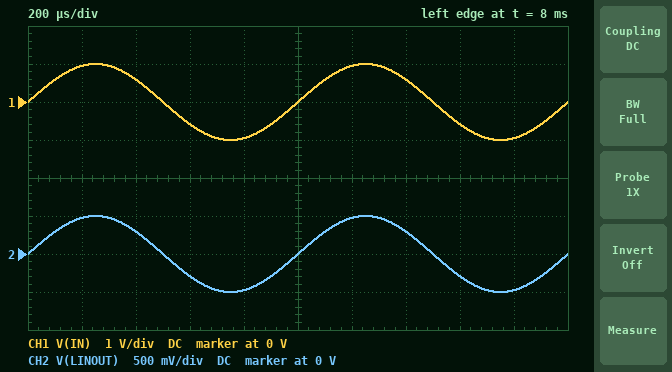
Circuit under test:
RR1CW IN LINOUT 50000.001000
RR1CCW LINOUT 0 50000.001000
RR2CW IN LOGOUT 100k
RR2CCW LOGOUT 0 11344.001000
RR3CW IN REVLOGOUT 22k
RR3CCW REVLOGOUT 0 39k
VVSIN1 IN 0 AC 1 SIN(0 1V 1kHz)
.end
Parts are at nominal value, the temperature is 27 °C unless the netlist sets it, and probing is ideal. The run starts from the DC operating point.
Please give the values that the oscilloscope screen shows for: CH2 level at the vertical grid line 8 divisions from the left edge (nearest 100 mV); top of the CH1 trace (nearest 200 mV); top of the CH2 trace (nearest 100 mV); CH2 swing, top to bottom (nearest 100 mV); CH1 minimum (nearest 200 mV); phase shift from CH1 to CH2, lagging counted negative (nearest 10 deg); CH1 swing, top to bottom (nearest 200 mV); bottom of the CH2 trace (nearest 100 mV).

-300 mV
1.0 V
500 mV
1.0 V
-1.0 V
0 deg
2.0 V
-500 mV
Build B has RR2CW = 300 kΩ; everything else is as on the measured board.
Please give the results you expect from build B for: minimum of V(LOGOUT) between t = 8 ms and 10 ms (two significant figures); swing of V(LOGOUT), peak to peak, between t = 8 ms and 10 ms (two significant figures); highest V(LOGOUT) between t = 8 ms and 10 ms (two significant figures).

-36 mV
73 mV
36 mV
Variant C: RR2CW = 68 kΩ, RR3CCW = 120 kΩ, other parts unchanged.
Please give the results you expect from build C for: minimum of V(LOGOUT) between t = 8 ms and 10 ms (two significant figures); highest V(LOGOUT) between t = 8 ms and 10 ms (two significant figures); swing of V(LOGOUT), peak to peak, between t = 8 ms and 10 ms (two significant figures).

-140 mV
140 mV
290 mV
